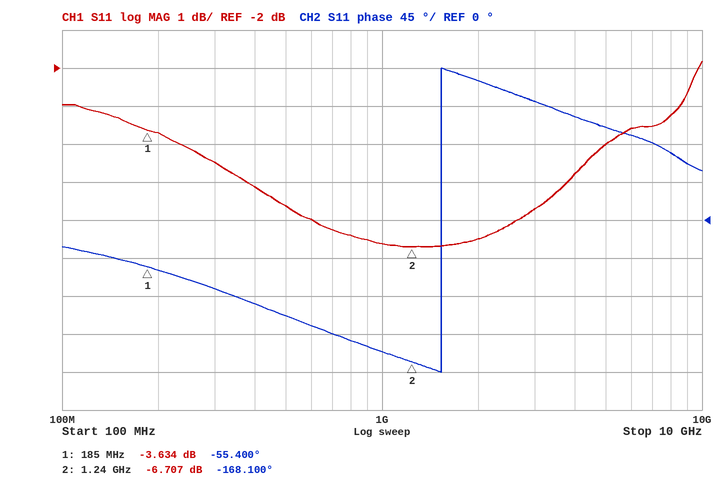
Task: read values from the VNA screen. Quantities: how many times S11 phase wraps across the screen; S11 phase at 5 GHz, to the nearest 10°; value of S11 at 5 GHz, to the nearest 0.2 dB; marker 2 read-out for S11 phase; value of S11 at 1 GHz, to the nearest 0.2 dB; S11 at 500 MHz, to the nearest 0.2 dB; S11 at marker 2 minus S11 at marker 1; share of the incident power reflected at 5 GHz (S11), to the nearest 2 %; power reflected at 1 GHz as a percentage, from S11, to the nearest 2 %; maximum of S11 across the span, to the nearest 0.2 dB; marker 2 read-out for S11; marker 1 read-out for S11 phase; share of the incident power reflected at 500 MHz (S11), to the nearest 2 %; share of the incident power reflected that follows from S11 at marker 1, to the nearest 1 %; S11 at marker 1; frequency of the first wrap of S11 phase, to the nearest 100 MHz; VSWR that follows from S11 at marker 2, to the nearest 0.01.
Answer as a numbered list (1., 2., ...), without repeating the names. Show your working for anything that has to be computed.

1. 1
2. 110°
3. -4.0 dB
4. -168.100°
5. -6.6 dB
6. -5.6 dB
7. -6.707 − (-3.634) = -3.073 dB
8. 10^(-4/10) ≈ 40 %
9. 10^(-6.6/10) ≈ 22 %
10. -1.8 dB
11. -6.707 dB
12. -55.400°
13. 10^(-5.6/10) ≈ 28 %
14. 10^(-3.634/10) ≈ 43 %
15. -3.634 dB
16. 1.5 GHz
17. (1 + 0.4620)/(1 − 0.4620) ≈ 2.72
